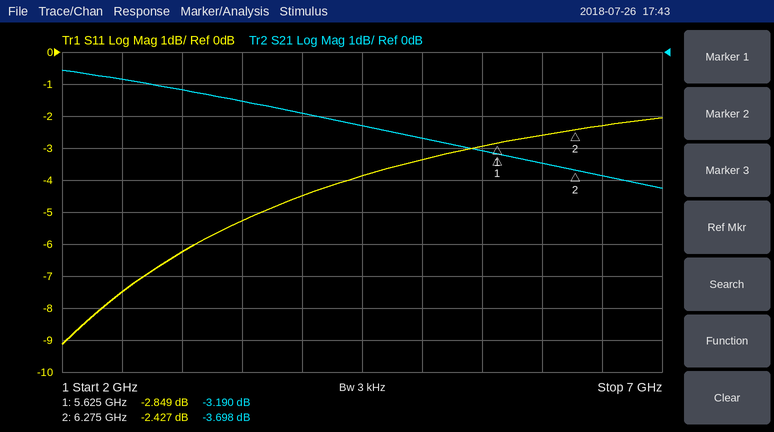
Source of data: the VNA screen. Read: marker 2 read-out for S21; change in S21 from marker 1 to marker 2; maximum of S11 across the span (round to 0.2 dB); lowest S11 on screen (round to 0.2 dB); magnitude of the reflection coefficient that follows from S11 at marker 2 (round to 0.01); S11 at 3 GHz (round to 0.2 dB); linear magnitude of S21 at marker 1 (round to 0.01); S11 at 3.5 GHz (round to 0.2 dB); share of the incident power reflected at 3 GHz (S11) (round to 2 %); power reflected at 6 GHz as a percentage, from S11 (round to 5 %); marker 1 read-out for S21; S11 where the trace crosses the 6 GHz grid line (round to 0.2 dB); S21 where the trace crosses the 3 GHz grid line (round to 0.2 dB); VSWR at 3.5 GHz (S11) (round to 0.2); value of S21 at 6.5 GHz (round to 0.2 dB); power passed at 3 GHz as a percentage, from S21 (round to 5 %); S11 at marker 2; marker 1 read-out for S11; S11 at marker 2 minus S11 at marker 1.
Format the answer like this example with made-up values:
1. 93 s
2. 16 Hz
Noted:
1. -3.698 dB
2. -0.508 dB
3. -2.0 dB
4. -9.2 dB
5. 0.76
6. -6.2 dB
7. 0.69
8. -5.2 dB
9. 24 %
10. 55 %
11. -3.190 dB
12. -2.6 dB
13. -1.2 dB
14. 3.4
15. -3.8 dB
16. 75 %
17. -2.427 dB
18. -2.849 dB
19. 0.422 dB
